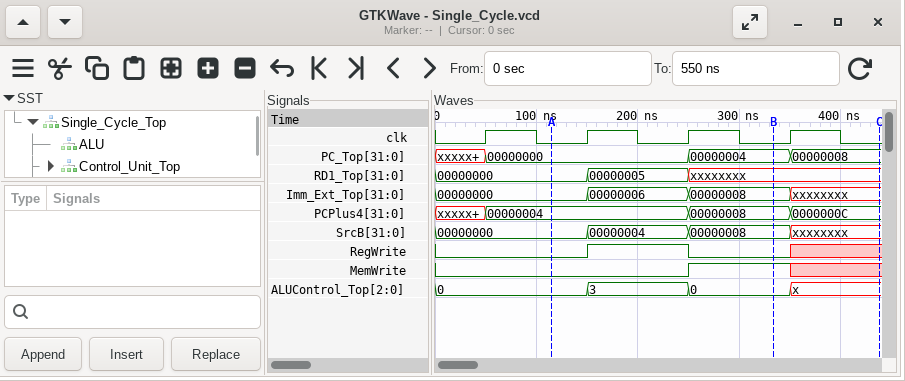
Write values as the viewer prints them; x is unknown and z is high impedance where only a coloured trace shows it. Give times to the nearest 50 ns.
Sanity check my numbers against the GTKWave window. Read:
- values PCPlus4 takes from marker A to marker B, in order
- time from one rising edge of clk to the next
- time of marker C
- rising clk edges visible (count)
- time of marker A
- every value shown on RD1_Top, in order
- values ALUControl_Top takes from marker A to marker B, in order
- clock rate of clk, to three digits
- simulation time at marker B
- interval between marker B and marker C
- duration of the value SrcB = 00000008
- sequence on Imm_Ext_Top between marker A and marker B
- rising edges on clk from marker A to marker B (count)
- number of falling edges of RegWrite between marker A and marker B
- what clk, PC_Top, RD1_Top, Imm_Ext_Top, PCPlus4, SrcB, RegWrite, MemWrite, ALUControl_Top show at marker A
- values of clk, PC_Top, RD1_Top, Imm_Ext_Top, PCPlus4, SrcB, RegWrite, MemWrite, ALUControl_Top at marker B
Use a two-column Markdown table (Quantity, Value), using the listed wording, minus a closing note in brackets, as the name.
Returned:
| Quantity | Value |
|---|---|
| values PCPlus4 takes from marker A to marker B, in order | 00000004, 00000008 |
| time from one rising edge of clk to the next | 100 ns |
| time of marker C | 450 ns |
| rising clk edges visible | 4 |
| time of marker A | 100 ns |
| every value shown on RD1_Top, in order | 00000000, 00000005, xxxxxxxx |
| values ALUControl_Top takes from marker A to marker B, in order | 0, 3, 0 |
| clock rate of clk, to three digits | 10.0 MHz |
| simulation time at marker B | 350 ns |
| interval between marker B and marker C | 100 ns |
| duration of the value SrcB = 00000008 | 100 ns |
| sequence on Imm_Ext_Top between marker A and marker B | 00000000, 00000006, 00000008 |
| rising edges on clk from marker A to marker B | 2 |
| number of falling edges of RegWrite between marker A and marker B | 1 |
| what clk, PC_Top, RD1_Top, Imm_Ext_Top, PCPlus4, SrcB, RegWrite, MemWrite, ALUControl_Top show at marker A | clk=0, PC_Top=00000000, RD1_Top=00000000, Imm_Ext_Top=00000000, PCPlus4=00000004, SrcB=00000000, RegWrite=0, MemWrite=0, ALUControl_Top=0 |
| values of clk, PC_Top, RD1_Top, Imm_Ext_Top, PCPlus4, SrcB, RegWrite, MemWrite, ALUControl_Top at marker B | clk=0, PC_Top=00000004, RD1_Top=xxxxxxxx, Imm_Ext_Top=00000008, PCPlus4=00000008, SrcB=00000008, RegWrite=0, MemWrite=1, ALUControl_Top=0 |
